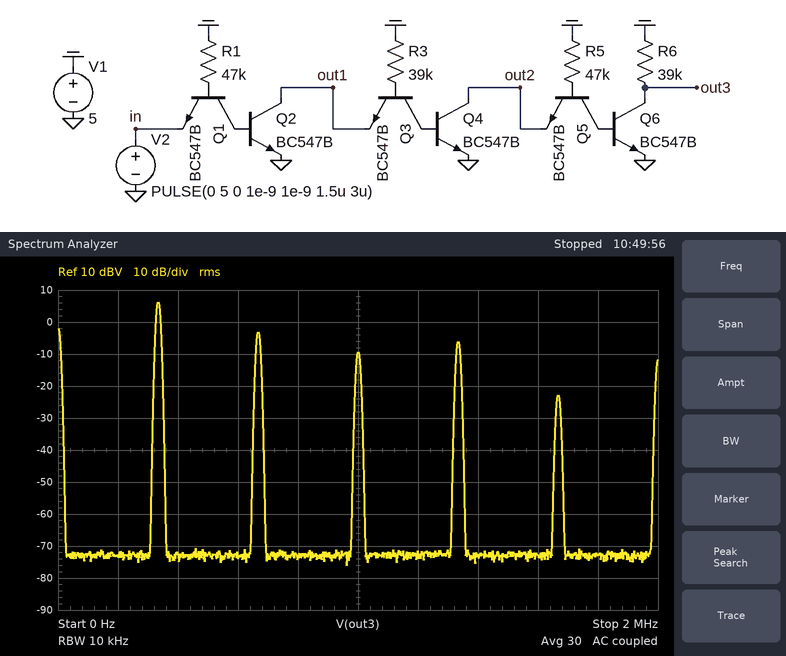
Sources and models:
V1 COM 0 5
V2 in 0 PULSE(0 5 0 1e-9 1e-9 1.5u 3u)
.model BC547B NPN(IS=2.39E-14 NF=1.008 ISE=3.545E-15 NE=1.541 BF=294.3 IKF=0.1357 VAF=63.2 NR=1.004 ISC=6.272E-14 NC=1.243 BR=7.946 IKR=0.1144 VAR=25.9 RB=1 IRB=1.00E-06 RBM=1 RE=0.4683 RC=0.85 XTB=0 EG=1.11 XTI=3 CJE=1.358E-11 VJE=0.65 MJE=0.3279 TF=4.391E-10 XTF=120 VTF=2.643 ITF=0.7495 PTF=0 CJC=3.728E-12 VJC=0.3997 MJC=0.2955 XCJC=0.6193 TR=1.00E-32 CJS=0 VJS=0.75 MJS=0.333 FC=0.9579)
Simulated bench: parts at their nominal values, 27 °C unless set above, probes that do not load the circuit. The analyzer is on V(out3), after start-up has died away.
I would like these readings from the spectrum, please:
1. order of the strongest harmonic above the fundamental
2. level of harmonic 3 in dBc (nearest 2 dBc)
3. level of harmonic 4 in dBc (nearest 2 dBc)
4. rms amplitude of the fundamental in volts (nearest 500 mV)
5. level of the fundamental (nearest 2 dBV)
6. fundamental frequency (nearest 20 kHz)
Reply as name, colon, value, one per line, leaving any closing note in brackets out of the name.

order of the strongest harmonic above the fundamental: 2
level of harmonic 3 in dBc: -16 dBc
level of harmonic 4 in dBc: -12 dBc
rms amplitude of the fundamental in volts: 2.0 V
level of the fundamental: 6 dBV
fundamental frequency: 340 kHz
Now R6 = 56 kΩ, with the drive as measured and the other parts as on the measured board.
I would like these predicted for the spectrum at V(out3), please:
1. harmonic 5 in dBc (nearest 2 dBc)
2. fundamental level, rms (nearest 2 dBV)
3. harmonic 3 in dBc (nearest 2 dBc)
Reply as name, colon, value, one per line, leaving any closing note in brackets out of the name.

harmonic 5 in dBc: -22 dBc
fundamental level, rms: 6 dBV
harmonic 3 in dBc: -18 dBc
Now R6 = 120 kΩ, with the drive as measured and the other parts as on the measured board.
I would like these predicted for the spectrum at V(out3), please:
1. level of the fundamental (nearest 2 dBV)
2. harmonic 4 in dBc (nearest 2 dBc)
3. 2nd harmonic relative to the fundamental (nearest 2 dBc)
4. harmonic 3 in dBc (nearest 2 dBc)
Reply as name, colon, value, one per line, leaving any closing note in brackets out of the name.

level of the fundamental: 4 dBV
harmonic 4 in dBc: -14 dBc
2nd harmonic relative to the fundamental: -6 dBc
harmonic 3 in dBc: -20 dBc
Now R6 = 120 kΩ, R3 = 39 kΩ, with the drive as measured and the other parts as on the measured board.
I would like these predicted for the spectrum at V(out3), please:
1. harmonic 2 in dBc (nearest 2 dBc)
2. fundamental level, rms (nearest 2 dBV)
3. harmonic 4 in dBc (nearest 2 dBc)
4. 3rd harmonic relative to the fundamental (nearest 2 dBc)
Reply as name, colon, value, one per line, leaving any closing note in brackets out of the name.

harmonic 2 in dBc: -6 dBc
fundamental level, rms: 4 dBV
harmonic 4 in dBc: -14 dBc
3rd harmonic relative to the fundamental: -20 dBc
